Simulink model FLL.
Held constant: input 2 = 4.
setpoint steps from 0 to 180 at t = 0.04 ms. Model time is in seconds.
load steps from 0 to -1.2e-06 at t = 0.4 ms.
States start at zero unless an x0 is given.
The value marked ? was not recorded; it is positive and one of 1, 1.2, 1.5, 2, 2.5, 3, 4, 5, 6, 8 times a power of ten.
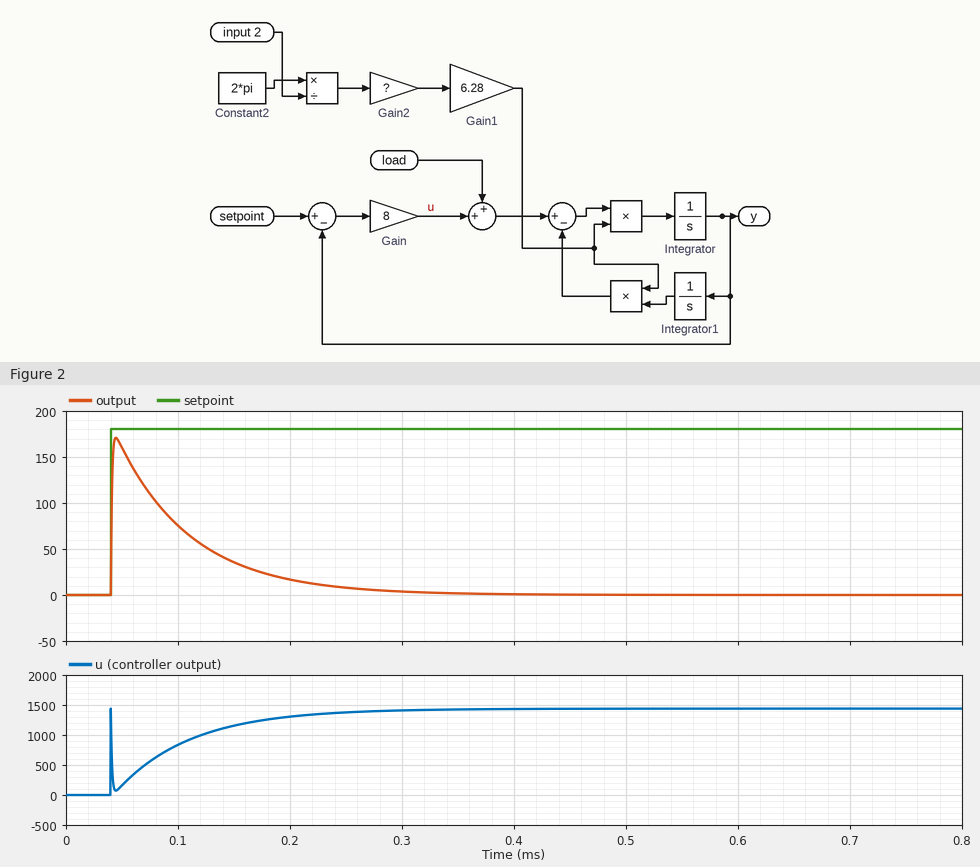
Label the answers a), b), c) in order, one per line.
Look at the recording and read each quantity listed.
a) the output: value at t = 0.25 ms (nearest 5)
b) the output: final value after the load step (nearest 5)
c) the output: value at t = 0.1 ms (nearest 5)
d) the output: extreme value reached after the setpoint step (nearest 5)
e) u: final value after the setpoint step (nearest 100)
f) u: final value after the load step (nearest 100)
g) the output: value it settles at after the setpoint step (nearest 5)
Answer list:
a) 10
b) 0
c) 75
d) 170
e) 1400
f) 1400
g) 0
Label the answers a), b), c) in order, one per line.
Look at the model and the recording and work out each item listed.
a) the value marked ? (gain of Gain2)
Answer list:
a) 12000
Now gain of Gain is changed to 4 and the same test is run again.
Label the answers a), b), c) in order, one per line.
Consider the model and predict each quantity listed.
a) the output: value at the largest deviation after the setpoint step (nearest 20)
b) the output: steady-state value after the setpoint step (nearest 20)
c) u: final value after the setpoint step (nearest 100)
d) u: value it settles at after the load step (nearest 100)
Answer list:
a) 160
b) 0
c) 700
d) 700
